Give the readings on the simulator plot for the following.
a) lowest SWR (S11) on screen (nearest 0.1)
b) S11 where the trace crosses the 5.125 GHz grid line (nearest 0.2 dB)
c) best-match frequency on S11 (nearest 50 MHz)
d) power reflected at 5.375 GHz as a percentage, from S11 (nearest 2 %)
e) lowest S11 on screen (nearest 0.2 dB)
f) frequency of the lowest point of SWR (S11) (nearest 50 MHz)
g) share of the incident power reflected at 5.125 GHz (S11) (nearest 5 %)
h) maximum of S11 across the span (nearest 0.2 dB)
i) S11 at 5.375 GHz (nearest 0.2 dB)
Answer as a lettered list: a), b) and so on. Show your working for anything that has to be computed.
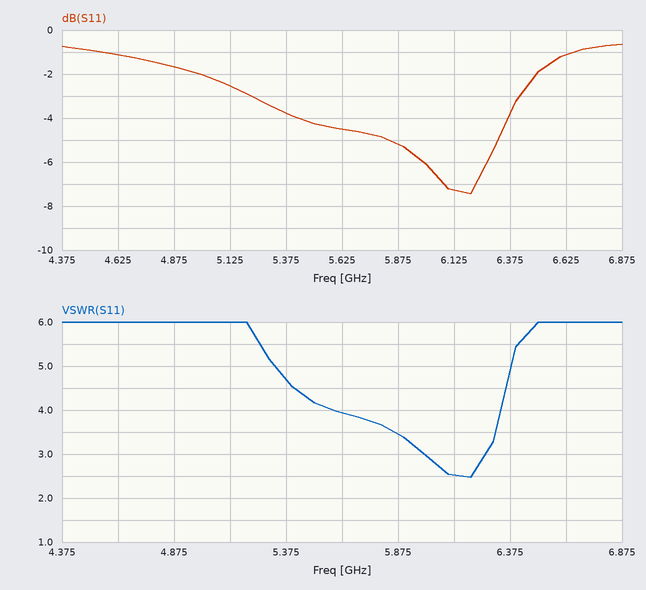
a) 2.5
b) -2.6 dB
c) 6.20 GHz
d) 10^(-3.8/10) ≈ 42 %
e) -7.4 dB
f) 6.20 GHz
g) 10^(-2.6/10) ≈ 55 %
h) -0.6 dB
i) -3.8 dB
